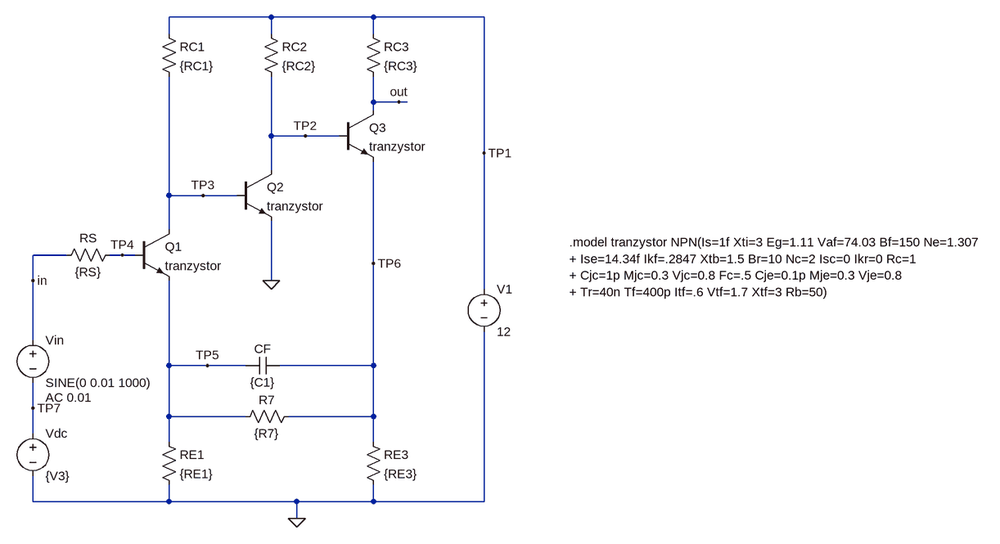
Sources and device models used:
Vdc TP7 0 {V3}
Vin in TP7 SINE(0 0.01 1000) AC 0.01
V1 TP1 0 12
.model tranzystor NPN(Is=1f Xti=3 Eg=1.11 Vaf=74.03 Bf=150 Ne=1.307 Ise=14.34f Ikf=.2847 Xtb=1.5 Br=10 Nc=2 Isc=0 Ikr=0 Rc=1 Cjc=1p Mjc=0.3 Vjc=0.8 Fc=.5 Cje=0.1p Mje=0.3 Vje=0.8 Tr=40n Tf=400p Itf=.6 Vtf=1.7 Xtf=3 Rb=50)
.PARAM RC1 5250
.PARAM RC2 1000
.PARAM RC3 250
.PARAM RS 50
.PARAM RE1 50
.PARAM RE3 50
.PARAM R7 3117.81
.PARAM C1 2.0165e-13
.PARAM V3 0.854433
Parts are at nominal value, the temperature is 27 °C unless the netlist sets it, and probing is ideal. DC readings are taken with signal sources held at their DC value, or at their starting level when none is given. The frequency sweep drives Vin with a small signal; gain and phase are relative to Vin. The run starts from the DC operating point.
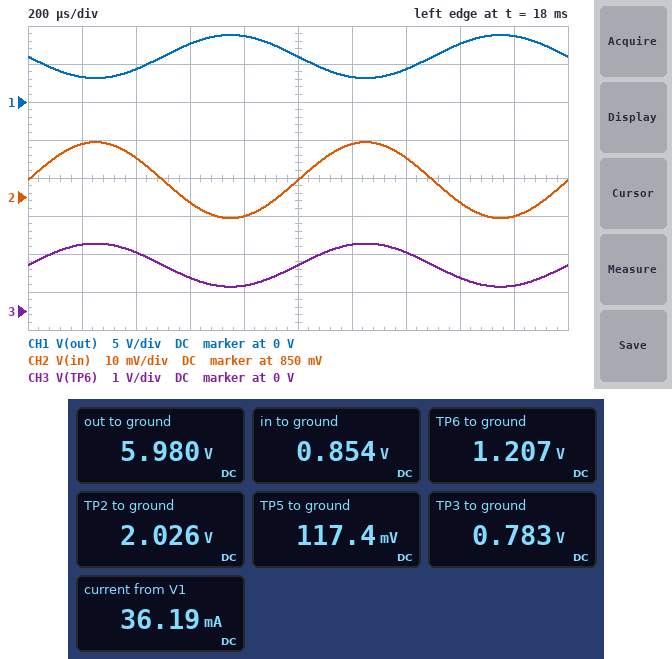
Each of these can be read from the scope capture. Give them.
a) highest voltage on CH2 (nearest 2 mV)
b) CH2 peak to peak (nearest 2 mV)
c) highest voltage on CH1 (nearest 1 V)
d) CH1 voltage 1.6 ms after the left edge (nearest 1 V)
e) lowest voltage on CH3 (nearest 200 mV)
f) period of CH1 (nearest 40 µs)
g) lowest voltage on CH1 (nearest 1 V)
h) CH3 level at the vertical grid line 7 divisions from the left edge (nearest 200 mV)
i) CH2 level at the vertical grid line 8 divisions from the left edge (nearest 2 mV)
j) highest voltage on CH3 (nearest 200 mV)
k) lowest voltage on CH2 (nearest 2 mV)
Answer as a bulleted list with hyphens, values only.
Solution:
- 864 mV
- 20 mV
- 9 V
- 8 V
- 600 mV
- 1.00 ms
- 3 V
- 1.6 V
- 848 mV
- 1.8 V
- 844 mV
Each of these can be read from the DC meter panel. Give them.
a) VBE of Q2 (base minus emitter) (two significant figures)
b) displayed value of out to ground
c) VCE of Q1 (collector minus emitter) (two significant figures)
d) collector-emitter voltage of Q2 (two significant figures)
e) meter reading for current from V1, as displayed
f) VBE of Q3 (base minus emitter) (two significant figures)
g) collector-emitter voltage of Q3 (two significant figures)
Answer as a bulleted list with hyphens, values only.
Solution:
- 780 mV
- 5.980 V
- 670 mV
- 2.0 V
- 36.19 mA
- 820 mV
- 4.8 V
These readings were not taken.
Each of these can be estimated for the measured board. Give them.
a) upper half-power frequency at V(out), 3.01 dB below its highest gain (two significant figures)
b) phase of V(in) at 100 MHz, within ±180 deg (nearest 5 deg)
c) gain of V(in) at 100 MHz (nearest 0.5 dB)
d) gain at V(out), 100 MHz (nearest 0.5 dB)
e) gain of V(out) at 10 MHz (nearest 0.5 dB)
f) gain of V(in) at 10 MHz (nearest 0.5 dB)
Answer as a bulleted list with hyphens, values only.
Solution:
- 35 MHz
- 0 deg
- 0 dB
- 28.5 dB
- 49.0 dB
- 0 dB
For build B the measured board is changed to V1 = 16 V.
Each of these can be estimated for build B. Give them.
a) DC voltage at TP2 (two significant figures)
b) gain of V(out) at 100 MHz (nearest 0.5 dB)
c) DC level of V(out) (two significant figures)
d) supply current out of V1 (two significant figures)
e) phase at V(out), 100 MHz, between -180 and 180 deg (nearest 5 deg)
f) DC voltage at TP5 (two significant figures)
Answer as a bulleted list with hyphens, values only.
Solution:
- 66 mV
- -59.0 dB
- 16 V
- 19 mA
- -135 deg
- 110 mV
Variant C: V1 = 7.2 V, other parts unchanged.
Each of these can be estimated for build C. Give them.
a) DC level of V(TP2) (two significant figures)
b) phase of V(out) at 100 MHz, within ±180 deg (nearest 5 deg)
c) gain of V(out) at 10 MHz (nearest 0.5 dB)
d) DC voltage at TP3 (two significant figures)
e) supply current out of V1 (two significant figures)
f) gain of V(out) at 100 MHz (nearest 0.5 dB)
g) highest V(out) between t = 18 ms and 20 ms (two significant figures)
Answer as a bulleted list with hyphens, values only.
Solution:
- 2.4 V
- 60 deg
- -48.0 dB
- 120 mV
- 29 mA
- -41.5 dB
- 1.4 V
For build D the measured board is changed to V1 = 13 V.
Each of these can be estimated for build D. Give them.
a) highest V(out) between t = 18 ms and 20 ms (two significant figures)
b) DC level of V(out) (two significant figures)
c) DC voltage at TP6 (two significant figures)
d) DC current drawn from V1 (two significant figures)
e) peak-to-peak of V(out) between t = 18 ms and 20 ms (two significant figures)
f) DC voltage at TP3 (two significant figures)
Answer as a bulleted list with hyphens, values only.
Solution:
- 13 V
- 10 V
- 570 mV
- 25 mA
- 5.6 V
- 790 mV
